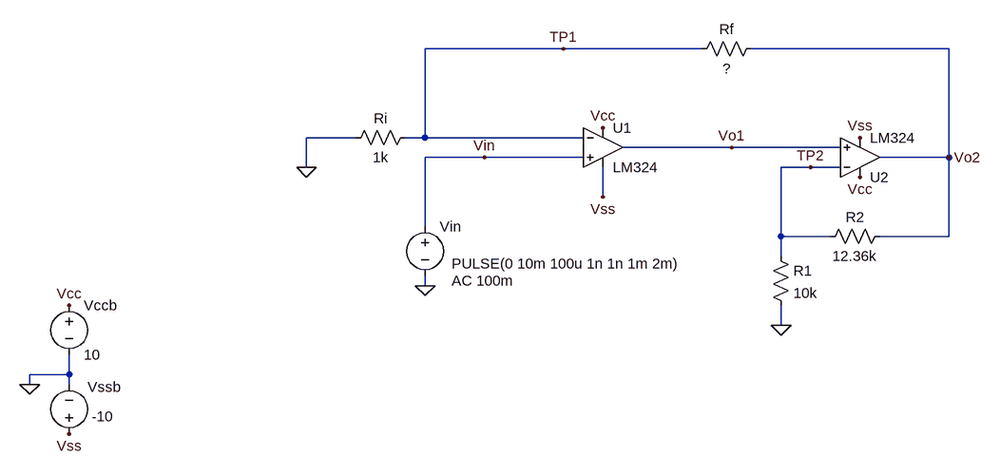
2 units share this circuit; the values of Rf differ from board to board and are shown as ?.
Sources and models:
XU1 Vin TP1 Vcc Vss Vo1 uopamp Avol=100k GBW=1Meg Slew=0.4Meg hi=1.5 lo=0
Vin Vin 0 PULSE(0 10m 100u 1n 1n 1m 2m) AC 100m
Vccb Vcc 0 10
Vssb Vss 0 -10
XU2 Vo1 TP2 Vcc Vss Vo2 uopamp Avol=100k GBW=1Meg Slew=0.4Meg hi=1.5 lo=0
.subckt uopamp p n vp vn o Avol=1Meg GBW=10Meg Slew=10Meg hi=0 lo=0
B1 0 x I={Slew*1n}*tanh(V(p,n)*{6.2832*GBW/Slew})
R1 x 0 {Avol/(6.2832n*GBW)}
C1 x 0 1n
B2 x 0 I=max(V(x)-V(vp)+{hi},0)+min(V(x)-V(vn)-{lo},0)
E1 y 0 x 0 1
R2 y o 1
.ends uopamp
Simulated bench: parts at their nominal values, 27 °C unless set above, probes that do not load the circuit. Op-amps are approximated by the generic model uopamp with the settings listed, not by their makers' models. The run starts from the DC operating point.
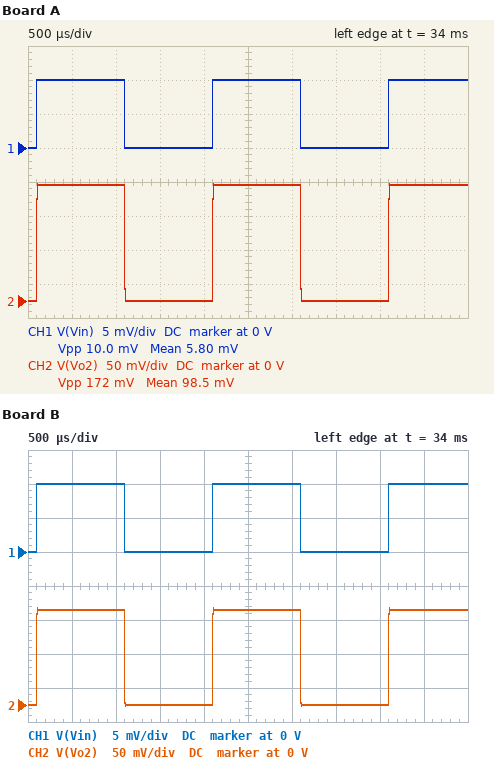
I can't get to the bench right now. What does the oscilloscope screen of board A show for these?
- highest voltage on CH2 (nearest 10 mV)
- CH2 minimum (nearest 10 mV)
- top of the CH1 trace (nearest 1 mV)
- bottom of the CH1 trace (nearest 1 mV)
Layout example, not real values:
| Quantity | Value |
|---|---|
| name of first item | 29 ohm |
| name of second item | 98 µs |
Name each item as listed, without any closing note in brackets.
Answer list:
| Quantity | Value |
|---|---|
| highest voltage on CH2 | 170 mV |
| CH2 minimum | 0 V |
| top of the CH1 trace | 10 mV |
| bottom of the CH1 trace | 0 V |
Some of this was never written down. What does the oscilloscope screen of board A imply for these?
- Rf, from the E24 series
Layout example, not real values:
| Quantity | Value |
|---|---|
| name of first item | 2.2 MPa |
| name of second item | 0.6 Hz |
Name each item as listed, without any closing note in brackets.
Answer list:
| Quantity | Value |
|---|---|
| Rf, from the E24 series | 16 kΩ |
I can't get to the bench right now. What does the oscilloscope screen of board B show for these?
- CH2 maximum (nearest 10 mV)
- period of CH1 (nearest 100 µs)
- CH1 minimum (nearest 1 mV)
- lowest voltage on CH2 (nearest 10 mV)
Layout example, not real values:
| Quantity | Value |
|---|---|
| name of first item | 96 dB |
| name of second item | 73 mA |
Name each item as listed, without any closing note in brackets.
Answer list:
| Quantity | Value |
|---|---|
| CH2 maximum | 140 mV |
| period of CH1 | 2.0 ms |
| CH1 minimum | 0 V |
| lowest voltage on CH2 | 0 V |
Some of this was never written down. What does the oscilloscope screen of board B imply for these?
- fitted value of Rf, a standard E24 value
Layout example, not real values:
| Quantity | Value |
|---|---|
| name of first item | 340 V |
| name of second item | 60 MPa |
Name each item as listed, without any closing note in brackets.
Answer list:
| Quantity | Value |
|---|---|
| fitted value of Rf, a standard E24 value | 13 kΩ |
